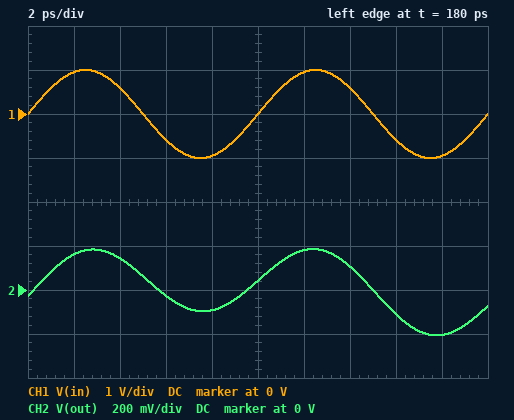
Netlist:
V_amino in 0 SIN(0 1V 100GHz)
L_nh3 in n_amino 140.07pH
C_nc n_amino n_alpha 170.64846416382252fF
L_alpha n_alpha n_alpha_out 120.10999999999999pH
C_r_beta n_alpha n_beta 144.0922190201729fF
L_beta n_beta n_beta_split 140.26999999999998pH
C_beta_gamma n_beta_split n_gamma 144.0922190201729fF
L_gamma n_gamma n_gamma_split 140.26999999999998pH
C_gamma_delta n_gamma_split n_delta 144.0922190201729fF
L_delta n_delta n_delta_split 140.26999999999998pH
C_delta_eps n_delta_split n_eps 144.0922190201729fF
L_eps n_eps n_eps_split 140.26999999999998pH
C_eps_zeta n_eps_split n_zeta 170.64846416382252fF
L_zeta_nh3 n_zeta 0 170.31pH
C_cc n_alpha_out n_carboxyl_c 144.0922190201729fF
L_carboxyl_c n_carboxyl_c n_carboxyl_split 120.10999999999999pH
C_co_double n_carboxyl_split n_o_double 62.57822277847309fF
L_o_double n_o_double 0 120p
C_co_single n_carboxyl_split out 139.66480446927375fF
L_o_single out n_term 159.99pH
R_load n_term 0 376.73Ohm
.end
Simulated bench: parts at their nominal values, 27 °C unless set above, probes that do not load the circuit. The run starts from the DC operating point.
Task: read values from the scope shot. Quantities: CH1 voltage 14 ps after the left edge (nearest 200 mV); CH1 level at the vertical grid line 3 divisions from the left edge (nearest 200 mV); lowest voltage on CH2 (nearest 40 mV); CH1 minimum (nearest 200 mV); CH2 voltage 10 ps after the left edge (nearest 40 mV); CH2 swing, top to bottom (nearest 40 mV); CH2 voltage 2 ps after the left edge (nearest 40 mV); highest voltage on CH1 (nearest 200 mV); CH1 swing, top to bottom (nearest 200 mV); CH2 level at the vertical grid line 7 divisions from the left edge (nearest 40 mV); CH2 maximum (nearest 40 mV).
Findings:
600 mV
-600 mV
-200 mV
-1.0 V
40 mV
400 mV
160 mV
1.0 V
2.0 V
120 mV
200 mV
